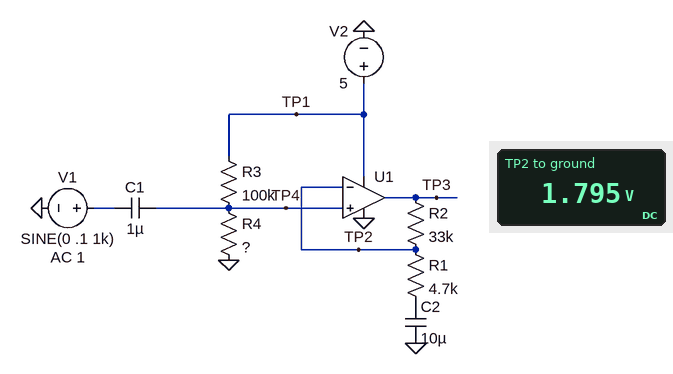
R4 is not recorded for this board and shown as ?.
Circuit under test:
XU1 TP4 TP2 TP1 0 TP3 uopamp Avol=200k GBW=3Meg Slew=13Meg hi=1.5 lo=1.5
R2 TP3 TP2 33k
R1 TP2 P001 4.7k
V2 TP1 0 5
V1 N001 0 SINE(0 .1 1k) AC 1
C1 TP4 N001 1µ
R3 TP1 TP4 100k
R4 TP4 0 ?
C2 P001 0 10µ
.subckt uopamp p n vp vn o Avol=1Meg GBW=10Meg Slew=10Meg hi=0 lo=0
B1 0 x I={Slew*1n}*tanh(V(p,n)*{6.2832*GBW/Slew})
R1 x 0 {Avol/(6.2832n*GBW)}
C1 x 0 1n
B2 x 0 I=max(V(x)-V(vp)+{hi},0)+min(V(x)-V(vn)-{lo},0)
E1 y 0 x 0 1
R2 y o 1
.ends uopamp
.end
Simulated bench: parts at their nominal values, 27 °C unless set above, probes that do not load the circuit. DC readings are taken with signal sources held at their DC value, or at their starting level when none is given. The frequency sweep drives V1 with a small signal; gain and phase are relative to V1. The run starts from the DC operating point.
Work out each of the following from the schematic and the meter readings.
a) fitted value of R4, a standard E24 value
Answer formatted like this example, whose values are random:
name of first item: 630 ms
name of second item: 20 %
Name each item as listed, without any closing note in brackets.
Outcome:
fitted value of R4, a standard E24 value: 56 kΩ
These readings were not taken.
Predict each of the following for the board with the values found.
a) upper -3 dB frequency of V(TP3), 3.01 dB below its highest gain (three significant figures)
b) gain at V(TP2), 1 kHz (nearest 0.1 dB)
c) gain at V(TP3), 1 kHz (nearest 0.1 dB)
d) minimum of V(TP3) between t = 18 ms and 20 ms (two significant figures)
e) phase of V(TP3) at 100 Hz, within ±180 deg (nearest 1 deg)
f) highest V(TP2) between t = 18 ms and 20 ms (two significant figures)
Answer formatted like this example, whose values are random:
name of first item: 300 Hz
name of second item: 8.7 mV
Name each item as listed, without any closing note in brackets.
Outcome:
upper -3 dB frequency of V(TP3), 3.01 dB below its highest gain: 374 kHz
gain at V(TP2), 1 kHz: 0 dB
gain at V(TP3), 1 kHz: 18.1 dB
minimum of V(TP3) between t = 18 ms and 20 ms: 1.5 V
phase of V(TP3) at 100 Hz, within ±180 deg: 4 deg
highest V(TP2) between t = 18 ms and 20 ms: 1.9 V
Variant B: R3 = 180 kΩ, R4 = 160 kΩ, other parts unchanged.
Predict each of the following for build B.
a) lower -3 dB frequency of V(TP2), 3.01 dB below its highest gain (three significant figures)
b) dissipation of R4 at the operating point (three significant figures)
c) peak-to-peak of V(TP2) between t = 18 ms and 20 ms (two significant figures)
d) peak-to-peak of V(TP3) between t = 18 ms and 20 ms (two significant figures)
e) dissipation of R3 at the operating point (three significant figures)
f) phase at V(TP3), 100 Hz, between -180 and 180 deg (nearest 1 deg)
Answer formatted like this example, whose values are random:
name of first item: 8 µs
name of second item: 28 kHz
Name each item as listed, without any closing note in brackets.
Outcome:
lower -3 dB frequency of V(TP2), 3.01 dB below its highest gain: 1.88 Hz
dissipation of R4 at the operating point: 34.6 µW
peak-to-peak of V(TP2) between t = 18 ms and 20 ms: 200 mV
peak-to-peak of V(TP3) between t = 18 ms and 20 ms: 1.6 V
dissipation of R3 at the operating point: 38.9 µW
phase at V(TP3), 100 Hz, between -180 and 180 deg: 3 deg
